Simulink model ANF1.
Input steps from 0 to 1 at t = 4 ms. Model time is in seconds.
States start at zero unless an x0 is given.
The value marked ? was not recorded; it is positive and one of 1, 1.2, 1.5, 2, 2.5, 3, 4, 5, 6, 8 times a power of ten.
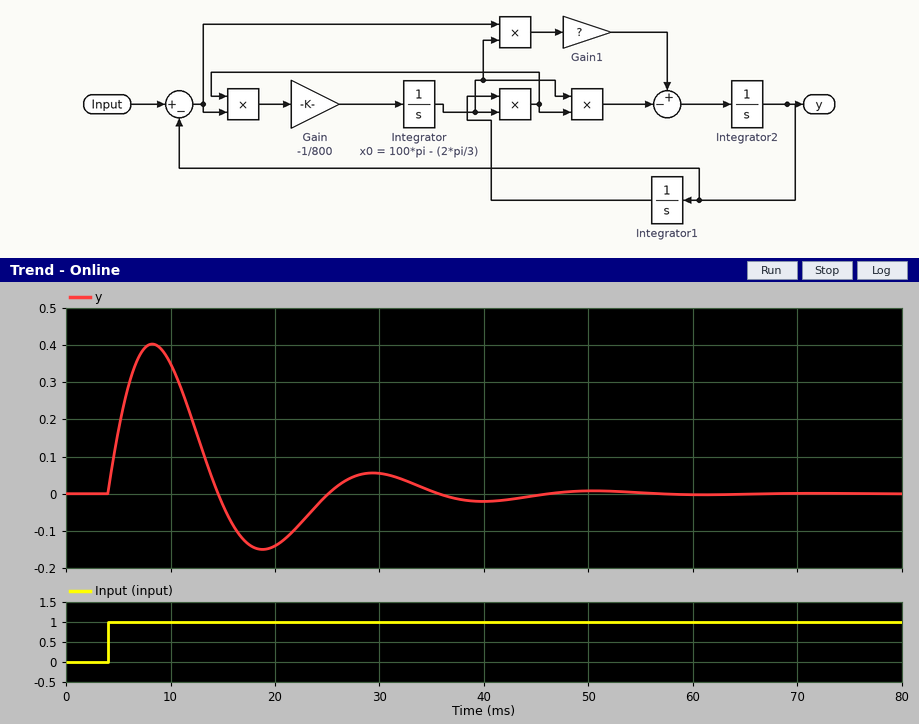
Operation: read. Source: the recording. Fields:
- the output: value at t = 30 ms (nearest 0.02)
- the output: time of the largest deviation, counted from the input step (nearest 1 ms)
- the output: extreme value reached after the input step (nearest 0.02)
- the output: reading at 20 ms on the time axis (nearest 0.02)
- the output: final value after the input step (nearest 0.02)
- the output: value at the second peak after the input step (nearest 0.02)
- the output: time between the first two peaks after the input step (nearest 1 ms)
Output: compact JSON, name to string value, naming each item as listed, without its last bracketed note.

{"the output: value at t = 30 ms": "0.06", "the output: time of the largest deviation, counted from the input step": "4 ms", "the output: extreme value reached after the input step": "0.40", "the output: reading at 20 ms on the time axis": "-0.14", "the output: final value after the input step": "0.00", "the output: value at the second peak after the input step": "0.06", "the output: time between the first two peaks after the input step": "21 ms"}
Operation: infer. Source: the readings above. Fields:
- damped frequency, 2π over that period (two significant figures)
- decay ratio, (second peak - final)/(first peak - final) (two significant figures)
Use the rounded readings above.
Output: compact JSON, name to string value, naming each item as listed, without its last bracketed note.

{"damped frequency, 2π over that period": "0.30 rad/ms", "decay ratio, (second peak - final)/(first peak - final)": "0.15"}
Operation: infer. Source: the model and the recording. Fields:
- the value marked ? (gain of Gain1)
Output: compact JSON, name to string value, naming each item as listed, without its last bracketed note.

{"the value marked ?": "0.6"}
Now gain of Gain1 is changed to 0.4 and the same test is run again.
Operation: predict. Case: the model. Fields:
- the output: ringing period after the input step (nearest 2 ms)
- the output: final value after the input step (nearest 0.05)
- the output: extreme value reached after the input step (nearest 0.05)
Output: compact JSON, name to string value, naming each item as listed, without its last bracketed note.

{"the output: ringing period after the input step": "20 ms", "the output: final value after the input step": "0.00", "the output: extreme value reached after the input step": "0.30"}
